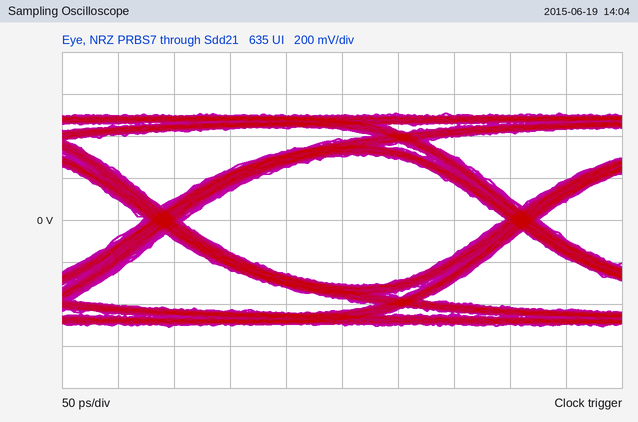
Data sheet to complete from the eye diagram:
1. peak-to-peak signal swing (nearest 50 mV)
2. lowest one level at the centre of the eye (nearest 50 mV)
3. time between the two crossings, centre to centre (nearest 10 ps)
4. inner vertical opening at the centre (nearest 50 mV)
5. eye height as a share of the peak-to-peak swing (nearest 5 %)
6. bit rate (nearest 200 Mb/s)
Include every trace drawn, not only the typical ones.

1.00 V
300 mV
320 ps
600 mV
60 %
3.2 Gb/s
